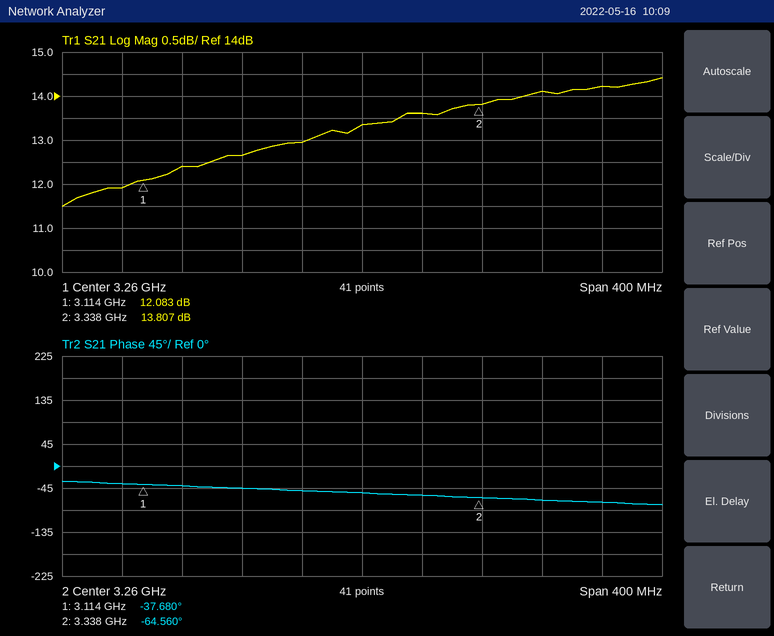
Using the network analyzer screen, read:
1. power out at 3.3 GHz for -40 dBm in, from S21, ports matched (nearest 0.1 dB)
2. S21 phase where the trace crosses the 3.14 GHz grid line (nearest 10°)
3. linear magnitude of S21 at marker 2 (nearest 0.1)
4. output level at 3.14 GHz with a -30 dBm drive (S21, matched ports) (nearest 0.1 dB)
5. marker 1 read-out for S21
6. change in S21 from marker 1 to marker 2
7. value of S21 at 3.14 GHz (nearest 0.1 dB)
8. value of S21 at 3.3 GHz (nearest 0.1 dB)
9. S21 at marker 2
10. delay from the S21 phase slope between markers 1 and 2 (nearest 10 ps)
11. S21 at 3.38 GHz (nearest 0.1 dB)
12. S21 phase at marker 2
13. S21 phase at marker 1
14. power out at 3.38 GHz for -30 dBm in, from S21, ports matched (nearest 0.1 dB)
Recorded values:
-26.4 dBm
-40°
4.9
-17.6 dBm
12.083 dB
1.724 dB
12.4 dB
13.6 dB
13.807 dB
330 ps
14.1 dB
-64.560°
-37.680°
-15.9 dBm
